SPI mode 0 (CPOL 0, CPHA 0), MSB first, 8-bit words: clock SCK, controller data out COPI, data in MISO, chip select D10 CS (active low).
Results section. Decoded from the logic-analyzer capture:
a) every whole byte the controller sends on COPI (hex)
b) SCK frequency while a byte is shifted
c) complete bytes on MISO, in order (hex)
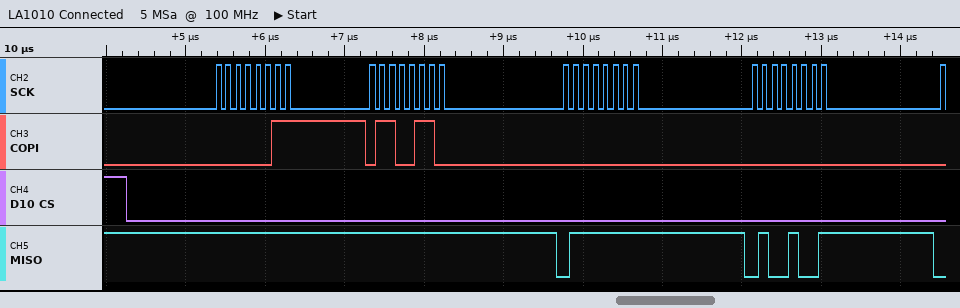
03 66 00 00
8 MHz
FF FF 7F 49
